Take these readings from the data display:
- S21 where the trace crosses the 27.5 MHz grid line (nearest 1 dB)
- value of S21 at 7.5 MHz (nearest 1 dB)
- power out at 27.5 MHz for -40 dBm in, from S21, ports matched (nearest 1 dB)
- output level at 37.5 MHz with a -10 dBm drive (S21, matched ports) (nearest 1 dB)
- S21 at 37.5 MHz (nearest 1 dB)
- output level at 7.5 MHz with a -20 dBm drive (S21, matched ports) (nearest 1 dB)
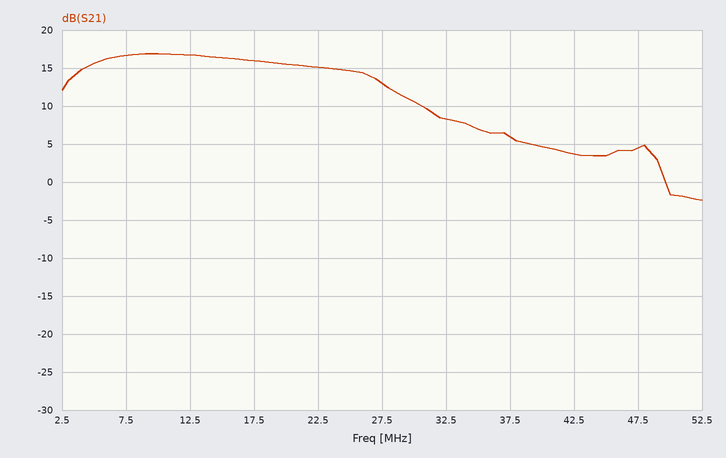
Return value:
13 dB
17 dB
-27 dBm
-4 dBm
6 dB
-3 dBm
